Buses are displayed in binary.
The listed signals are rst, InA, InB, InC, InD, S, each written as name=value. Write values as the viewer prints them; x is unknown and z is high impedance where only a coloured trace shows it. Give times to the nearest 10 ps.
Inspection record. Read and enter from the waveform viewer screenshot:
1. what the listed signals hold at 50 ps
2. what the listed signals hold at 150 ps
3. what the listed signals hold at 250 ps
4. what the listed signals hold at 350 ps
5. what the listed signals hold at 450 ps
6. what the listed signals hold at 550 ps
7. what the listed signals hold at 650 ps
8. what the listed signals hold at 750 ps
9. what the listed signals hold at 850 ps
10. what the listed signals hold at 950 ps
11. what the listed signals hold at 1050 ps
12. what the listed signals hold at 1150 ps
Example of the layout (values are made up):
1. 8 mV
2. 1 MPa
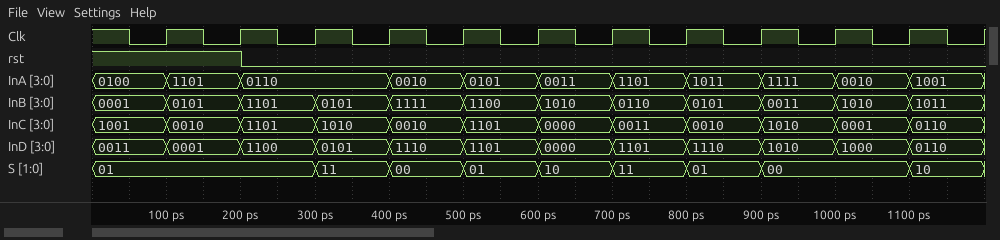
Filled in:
1. rst=1, InA=0100, InB=0001, InC=1001, InD=0011, S=01
2. rst=1, InA=1101, InB=0101, InC=0010, InD=0001, S=01
3. rst=0, InA=0110, InB=1101, InC=1101, InD=1100, S=01
4. rst=0, InA=0110, InB=0101, InC=1010, InD=0101, S=11
5. rst=0, InA=0010, InB=1111, InC=0010, InD=1110, S=00
6. rst=0, InA=0101, InB=1100, InC=1101, InD=1101, S=01
7. rst=0, InA=0011, InB=1010, InC=0000, InD=0000, S=10
8. rst=0, InA=1101, InB=0110, InC=0011, InD=1101, S=11
9. rst=0, InA=1011, InB=0101, InC=0010, InD=1110, S=01
10. rst=0, InA=1111, InB=0011, InC=1010, InD=1010, S=00
11. rst=0, InA=0010, InB=1010, InC=0001, InD=1000, S=00
12. rst=0, InA=1001, InB=1011, InC=0110, InD=0110, S=10
